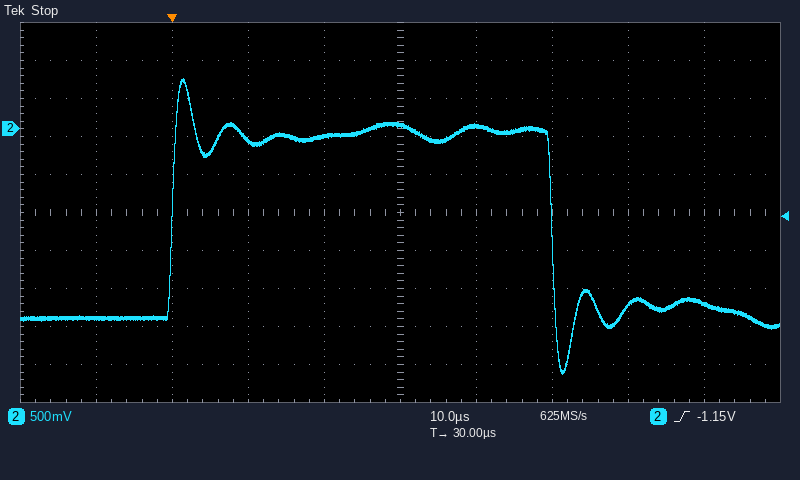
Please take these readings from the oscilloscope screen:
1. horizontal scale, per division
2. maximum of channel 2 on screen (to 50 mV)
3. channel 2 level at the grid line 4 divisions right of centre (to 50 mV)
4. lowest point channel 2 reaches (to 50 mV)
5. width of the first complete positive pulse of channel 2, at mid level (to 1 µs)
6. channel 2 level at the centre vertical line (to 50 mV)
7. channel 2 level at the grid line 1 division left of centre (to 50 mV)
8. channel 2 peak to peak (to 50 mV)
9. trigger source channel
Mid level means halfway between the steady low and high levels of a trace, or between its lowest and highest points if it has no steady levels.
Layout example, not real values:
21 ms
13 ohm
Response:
10 µs
650 mV
-2.30 V
-3.25 V
50 µs
50 mV
-100 mV
3.90 V
channel 2
